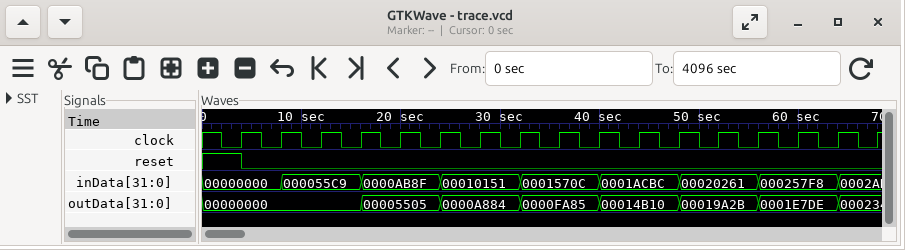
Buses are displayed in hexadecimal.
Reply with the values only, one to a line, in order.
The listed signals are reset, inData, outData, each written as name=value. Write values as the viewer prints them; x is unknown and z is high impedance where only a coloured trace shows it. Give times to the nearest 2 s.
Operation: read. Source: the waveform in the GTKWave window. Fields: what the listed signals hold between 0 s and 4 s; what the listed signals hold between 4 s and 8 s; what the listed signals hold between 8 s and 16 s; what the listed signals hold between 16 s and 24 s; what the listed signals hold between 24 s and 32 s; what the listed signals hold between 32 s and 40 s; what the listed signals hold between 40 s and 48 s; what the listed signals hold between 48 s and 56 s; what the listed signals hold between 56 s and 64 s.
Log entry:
reset=1, inData=00000000, outData=00000000
reset=0, inData=00000000, outData=00000000
reset=0, inData=000055C9, outData=00000000
reset=0, inData=0000AB8F, outData=00005505
reset=0, inData=00010151, outData=0000A884
reset=0, inData=0001570C, outData=0000FA85
reset=0, inData=0001ACBC, outData=00014B10
reset=0, inData=00020261, outData=00019A2B
reset=0, inData=000257F8, outData=0001E7DE
